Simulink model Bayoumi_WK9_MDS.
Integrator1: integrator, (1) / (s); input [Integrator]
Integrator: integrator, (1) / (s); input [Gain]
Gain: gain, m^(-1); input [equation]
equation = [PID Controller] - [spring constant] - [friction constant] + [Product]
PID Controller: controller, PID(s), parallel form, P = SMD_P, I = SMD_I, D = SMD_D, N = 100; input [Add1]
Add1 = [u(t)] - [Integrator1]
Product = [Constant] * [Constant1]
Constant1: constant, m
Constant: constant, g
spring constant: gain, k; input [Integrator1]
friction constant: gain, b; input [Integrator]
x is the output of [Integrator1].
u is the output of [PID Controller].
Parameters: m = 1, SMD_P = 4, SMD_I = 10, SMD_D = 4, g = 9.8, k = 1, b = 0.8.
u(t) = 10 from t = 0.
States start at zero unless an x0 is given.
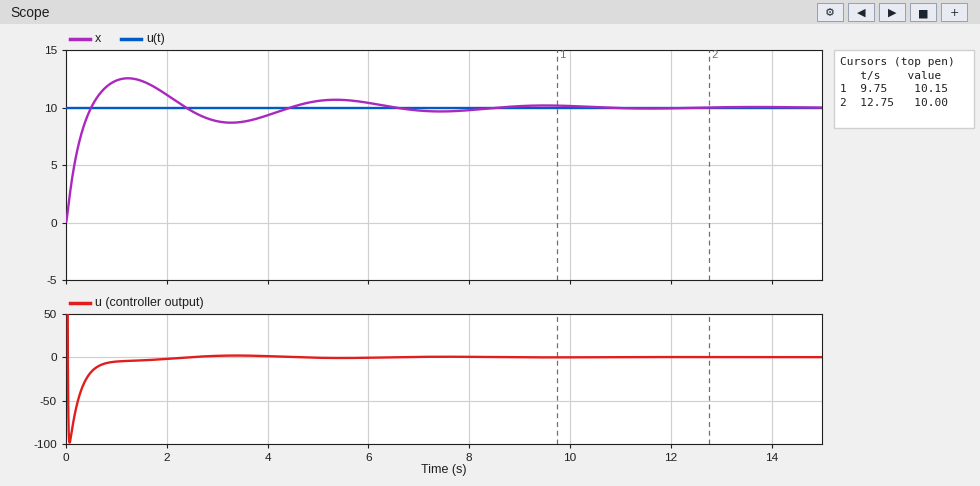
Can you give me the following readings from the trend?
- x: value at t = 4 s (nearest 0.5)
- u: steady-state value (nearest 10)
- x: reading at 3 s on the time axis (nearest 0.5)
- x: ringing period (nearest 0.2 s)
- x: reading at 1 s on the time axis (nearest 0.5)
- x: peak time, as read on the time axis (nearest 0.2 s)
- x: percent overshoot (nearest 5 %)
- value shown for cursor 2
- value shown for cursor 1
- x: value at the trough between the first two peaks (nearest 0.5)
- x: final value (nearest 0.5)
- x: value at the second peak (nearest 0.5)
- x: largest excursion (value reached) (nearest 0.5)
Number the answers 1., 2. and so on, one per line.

1. 9.5
2. 0
3. 9.0
4. 4.2 s
5. 12.5
6. 1.2 s
7. 25 %
8. 10.00
9. 10.15
10. 8.5
11. 10.0
12. 10.5
13. 12.5
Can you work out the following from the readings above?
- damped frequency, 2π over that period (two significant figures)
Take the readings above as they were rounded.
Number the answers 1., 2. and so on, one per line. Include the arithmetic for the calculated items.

1. 2π / 4.2 = 1.5 rad/s
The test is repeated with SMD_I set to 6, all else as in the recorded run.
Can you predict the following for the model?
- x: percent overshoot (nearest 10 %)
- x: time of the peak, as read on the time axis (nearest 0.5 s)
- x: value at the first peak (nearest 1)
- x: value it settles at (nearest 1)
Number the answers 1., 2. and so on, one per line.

1. 20 %
2. 1.5 s
3. 12
4. 10
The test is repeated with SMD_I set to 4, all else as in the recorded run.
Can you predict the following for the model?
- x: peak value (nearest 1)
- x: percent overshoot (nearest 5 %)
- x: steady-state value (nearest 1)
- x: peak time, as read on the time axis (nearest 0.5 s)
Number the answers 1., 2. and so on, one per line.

1. 11
2. 15 %
3. 10
4. 1.5 s
